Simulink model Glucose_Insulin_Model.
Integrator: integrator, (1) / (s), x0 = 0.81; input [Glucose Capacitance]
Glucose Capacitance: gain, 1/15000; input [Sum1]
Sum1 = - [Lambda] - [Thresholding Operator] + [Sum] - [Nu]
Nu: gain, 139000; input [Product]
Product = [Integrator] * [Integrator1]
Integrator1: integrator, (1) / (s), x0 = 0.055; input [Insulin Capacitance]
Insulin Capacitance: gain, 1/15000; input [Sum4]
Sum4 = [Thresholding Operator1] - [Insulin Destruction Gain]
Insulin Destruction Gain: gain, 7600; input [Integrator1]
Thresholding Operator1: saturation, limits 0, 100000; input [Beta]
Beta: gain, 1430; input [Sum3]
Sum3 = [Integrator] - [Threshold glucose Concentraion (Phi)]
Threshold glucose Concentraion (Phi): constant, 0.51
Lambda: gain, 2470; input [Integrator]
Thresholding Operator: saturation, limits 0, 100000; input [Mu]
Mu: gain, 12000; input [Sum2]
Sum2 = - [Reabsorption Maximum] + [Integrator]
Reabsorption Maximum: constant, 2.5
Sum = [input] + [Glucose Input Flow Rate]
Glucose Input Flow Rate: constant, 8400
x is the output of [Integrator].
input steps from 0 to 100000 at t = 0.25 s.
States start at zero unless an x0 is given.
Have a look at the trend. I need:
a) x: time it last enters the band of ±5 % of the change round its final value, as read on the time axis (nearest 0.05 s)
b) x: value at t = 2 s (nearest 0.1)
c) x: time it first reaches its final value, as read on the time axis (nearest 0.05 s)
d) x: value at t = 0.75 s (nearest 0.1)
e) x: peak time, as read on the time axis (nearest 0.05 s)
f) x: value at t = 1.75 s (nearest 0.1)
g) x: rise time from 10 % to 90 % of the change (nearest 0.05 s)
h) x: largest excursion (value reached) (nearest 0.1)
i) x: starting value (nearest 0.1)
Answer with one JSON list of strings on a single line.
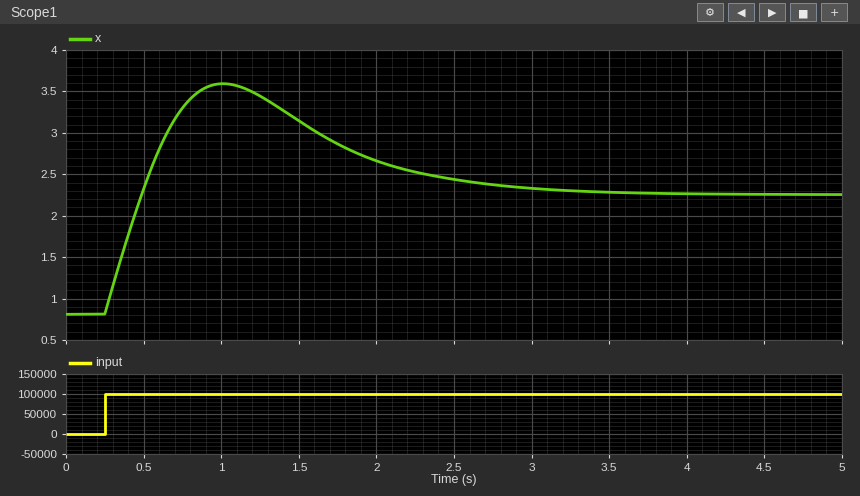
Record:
["3.05 s", "2.7", "0.50 s", "3.3", "1.00 s", "2.9", "0.20 s", "3.6", "0.8"]
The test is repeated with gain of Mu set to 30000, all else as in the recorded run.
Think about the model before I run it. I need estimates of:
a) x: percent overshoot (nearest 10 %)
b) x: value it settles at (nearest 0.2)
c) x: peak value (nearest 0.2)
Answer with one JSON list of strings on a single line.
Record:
["80 %", "2.2", "3.4"]
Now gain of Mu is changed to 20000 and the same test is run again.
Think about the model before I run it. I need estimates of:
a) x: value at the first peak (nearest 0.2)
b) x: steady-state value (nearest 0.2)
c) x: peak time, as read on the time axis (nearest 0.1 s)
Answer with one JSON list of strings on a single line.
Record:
["3.4", "2.2", "1.0 s"]
